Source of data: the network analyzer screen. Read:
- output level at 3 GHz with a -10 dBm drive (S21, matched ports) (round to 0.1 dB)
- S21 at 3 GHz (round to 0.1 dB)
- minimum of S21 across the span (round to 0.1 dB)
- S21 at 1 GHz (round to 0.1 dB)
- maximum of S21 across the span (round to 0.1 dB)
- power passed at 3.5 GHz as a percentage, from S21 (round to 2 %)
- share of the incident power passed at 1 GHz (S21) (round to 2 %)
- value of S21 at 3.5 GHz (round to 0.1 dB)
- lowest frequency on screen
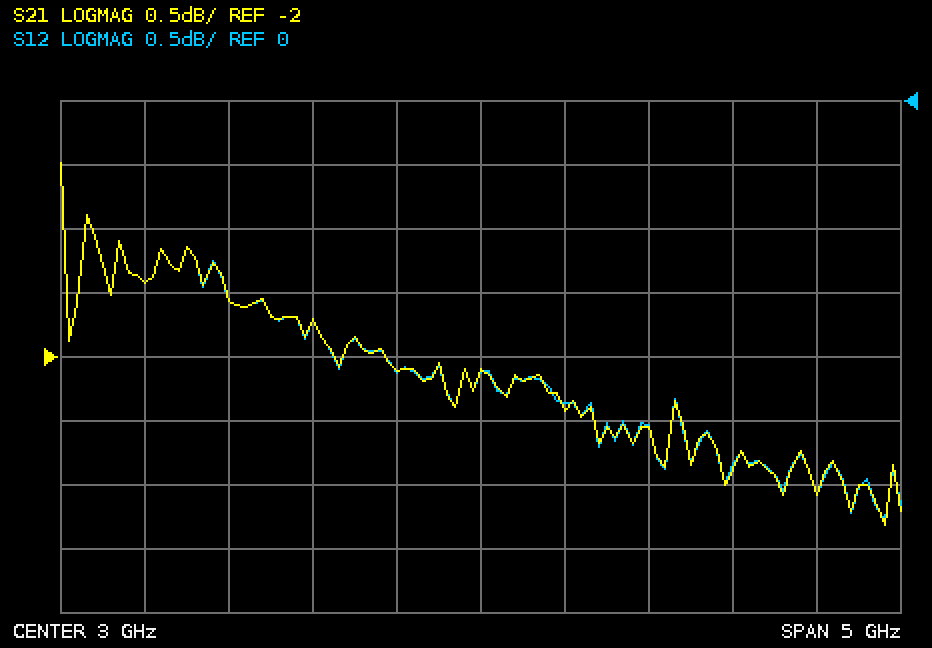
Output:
-12.1 dBm
-2.1 dB
-3.3 dB
-1.4 dB
-0.5 dB
58 %
72 %
-2.4 dB
500 MHz
